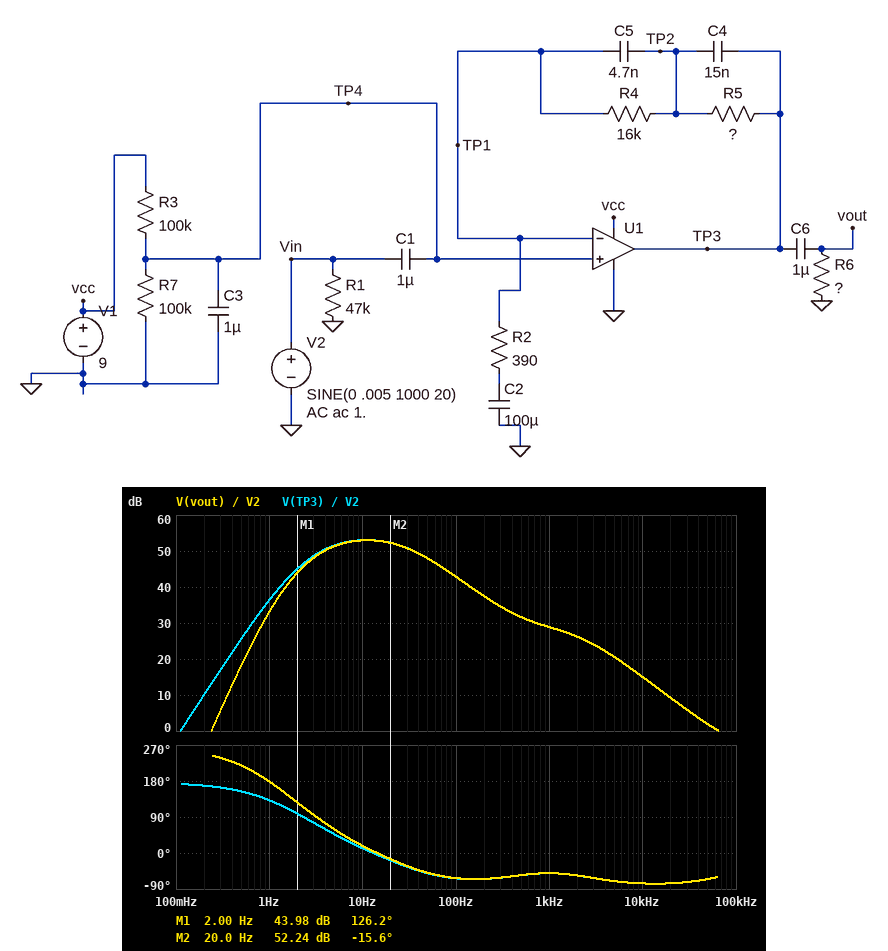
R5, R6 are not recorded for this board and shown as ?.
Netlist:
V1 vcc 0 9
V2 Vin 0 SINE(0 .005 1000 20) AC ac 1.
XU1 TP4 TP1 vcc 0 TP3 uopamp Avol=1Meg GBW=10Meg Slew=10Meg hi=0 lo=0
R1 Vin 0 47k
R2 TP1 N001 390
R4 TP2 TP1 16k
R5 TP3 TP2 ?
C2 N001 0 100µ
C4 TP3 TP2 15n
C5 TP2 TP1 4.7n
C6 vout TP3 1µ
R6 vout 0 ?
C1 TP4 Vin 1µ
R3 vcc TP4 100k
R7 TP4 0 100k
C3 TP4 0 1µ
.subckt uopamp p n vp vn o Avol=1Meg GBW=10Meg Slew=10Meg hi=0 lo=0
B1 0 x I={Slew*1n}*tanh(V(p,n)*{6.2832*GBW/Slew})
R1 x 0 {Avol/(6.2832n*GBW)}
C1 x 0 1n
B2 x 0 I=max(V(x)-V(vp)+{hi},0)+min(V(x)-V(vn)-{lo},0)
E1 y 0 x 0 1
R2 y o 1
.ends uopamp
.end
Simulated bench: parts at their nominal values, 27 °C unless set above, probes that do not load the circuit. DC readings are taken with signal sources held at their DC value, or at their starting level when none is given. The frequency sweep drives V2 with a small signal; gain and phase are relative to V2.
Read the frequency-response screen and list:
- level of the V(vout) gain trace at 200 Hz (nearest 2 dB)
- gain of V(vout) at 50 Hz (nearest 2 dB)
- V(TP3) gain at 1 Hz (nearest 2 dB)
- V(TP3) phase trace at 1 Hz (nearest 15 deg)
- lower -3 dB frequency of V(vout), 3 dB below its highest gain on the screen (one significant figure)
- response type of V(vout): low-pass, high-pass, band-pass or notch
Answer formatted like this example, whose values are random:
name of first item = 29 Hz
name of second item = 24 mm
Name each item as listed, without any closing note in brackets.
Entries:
level of the V(vout) gain trace at 200 Hz = 38 dB
gain of V(vout) at 50 Hz = 48 dB
V(TP3) gain at 1 Hz = 36 dB
V(TP3) phase trace at 1 Hz = 135 deg
lower -3 dB frequency of V(vout), 3 dB below its highest gain on the screen = 4 Hz
response type of V(vout): low-pass, high-pass, band-pass or notch = band-pass
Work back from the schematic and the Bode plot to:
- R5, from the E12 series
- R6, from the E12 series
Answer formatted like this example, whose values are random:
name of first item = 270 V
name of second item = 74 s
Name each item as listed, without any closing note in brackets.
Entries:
R5, from the E12 series = 390 kΩ
R6, from the E12 series = 150 kΩ
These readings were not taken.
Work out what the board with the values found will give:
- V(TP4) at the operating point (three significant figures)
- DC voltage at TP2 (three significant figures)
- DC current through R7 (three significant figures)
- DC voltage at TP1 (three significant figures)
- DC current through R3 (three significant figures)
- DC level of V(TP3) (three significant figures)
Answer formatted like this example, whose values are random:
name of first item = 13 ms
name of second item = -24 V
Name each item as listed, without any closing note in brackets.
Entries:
V(TP4) at the operating point = 4.50 V
DC voltage at TP2 = 4.50 V
DC current through R7 = 45.0 µA
DC voltage at TP1 = 4.50 V
DC current through R3 = 45.0 µA
DC level of V(TP3) = 4.50 V
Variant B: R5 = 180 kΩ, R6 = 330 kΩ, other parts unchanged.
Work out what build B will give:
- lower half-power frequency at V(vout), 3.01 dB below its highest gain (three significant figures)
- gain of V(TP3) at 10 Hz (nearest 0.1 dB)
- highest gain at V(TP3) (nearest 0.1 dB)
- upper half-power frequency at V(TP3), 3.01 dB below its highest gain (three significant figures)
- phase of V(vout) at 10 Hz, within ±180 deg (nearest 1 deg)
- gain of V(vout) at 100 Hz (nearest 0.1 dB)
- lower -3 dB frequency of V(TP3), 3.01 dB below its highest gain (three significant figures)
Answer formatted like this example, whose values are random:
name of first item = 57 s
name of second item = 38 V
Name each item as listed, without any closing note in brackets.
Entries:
lower half-power frequency at V(vout), 3.01 dB below its highest gain = 4.13 Hz
gain of V(TP3) at 10 Hz = 47.1 dB
highest gain at V(TP3) = 47.4 dB
upper half-power frequency at V(TP3), 3.01 dB below its highest gain = 67.9 Hz
phase of V(vout) at 10 Hz, within ±180 deg = 25 deg
gain of V(vout) at 100 Hz = 42.2 dB
lower -3 dB frequency of V(TP3), 3.01 dB below its highest gain = 4.09 Hz
